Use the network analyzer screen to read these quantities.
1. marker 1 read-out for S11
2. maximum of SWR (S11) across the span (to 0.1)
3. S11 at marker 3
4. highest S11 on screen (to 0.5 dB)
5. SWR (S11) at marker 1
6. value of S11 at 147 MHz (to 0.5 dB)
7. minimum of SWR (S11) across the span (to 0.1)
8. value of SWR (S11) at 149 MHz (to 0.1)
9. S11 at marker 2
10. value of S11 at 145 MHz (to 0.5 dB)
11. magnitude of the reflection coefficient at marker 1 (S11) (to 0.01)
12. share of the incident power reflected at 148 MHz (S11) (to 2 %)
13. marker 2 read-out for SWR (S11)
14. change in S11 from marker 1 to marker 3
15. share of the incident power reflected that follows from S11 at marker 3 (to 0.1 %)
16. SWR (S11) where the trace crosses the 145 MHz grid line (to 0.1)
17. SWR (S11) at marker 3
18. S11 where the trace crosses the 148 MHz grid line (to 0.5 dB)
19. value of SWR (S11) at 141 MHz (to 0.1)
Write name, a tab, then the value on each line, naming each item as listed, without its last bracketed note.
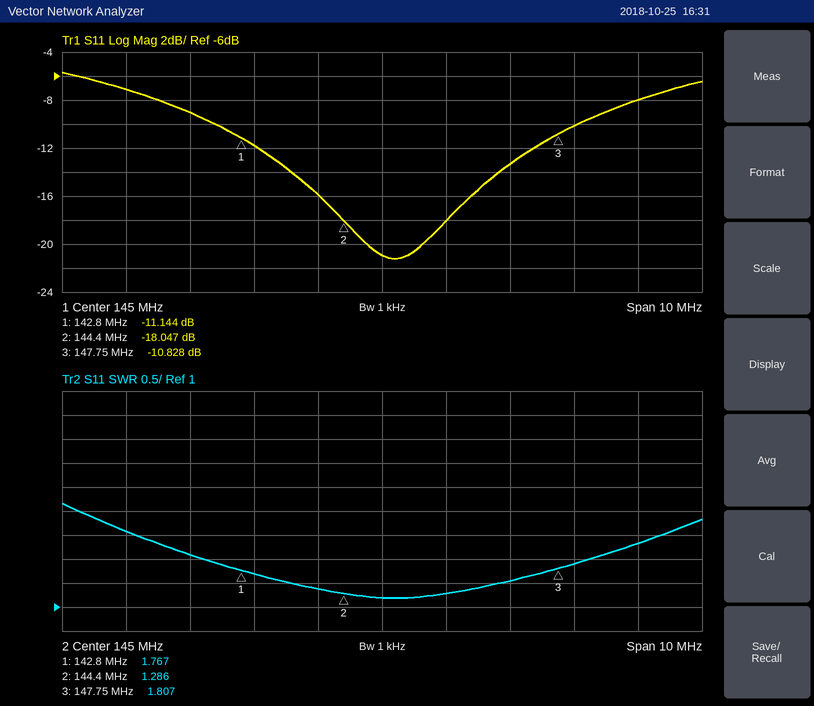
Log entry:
marker 1 read-out for S11	-11.144 dB
maximum of SWR (S11) across the span	3.2
S11 at marker 3	-10.828 dB
highest S11 on screen	-5.5 dB
SWR (S11) at marker 1	1.767
value of S11 at 147 MHz	-13.5 dB
minimum of SWR (S11) across the span	1.2
value of SWR (S11) at 149 MHz	2.3
S11 at marker 2	-18.047 dB
value of S11 at 145 MHz	-21.0 dB
magnitude of the reflection coefficient at marker 1 (S11)	0.28
share of the incident power reflected at 148 MHz (S11)	10 %
marker 2 read-out for SWR	1.286
change in S11 from marker 1 to marker 3	0.316 dB
share of the incident power reflected that follows from S11 at marker 3	8.3 %
SWR (S11) where the trace crosses the 145 MHz grid line	1.2
SWR (S11) at marker 3	1.807
S11 where the trace crosses the 148 MHz grid line	-10.0 dB
value of SWR (S11) at 141 MHz	2.6
